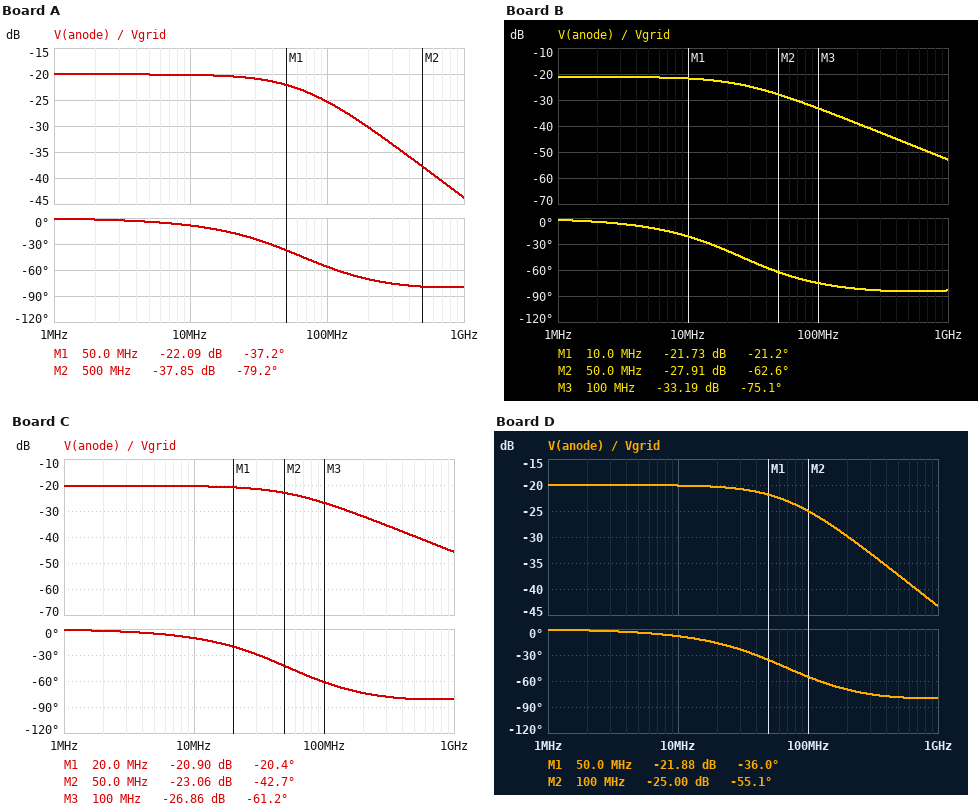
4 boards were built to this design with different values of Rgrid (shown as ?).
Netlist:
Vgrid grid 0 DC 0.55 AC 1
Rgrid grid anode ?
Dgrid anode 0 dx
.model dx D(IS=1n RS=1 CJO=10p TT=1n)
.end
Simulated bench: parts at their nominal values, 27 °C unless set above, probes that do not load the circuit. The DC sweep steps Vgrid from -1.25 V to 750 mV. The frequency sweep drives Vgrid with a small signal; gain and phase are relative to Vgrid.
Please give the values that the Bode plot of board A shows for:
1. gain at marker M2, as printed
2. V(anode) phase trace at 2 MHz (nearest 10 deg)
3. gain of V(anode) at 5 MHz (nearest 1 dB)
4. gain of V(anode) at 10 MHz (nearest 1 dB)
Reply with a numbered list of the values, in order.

1. -37.85 dB
2. 0 deg
3. -20 dB
4. -20 dB
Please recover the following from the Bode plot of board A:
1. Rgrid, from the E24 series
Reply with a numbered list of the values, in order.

1. 1.3 kΩ
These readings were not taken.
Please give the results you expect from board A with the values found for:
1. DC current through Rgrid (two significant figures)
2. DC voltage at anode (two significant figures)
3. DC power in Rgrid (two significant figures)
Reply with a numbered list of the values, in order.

1. 180 µA
2. 310 mV
3. 43 µW
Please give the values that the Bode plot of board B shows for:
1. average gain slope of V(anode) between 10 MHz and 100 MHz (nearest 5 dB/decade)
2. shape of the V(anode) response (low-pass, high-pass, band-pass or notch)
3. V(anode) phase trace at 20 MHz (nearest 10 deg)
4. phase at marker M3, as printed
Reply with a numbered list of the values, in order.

1. -10 dB/decade
2. low-pass
3. -40 deg
4. -75.1 deg
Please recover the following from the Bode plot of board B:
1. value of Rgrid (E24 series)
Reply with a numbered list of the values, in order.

1. 5.1 kΩ
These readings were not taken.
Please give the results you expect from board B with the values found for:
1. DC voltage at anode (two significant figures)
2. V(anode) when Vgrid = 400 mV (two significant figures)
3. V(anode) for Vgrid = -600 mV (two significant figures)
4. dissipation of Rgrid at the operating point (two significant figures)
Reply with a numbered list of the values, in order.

1. 280 mV
2. 260 mV
3. -600 mV
4. 14 µW
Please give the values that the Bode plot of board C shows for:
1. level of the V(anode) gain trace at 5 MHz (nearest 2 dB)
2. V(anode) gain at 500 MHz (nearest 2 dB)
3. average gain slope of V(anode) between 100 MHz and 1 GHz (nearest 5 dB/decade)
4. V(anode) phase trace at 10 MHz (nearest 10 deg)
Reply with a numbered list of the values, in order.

1. -20 dB
2. -40 dB
3. -20 dB/decade
4. -10 deg
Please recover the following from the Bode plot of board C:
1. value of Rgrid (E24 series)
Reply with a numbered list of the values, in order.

1. 1.8 kΩ
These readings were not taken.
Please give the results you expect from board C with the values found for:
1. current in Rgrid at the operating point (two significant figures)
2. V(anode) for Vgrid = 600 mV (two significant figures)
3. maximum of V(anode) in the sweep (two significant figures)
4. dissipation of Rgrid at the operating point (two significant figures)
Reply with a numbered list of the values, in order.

1. 140 µA
2. 310 mV
3. 320 mV
4. 33 µW
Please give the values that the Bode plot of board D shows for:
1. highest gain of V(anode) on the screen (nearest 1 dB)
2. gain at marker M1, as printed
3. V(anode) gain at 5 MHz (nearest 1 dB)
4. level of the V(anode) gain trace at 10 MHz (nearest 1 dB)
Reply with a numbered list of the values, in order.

1. -20 dB
2. -21.88 dB
3. -20 dB
4. -20 dB
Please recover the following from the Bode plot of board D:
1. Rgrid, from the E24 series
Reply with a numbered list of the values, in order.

1. 1.2 kΩ
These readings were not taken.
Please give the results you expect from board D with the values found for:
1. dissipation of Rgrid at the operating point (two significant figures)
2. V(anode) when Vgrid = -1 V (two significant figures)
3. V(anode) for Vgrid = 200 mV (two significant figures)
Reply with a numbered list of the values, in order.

1. 46 µW
2. -1.0 V
3. 200 mV
